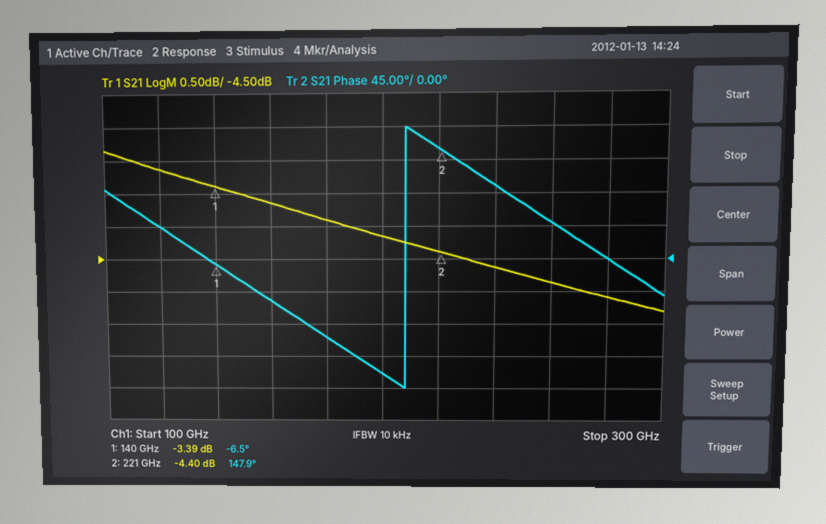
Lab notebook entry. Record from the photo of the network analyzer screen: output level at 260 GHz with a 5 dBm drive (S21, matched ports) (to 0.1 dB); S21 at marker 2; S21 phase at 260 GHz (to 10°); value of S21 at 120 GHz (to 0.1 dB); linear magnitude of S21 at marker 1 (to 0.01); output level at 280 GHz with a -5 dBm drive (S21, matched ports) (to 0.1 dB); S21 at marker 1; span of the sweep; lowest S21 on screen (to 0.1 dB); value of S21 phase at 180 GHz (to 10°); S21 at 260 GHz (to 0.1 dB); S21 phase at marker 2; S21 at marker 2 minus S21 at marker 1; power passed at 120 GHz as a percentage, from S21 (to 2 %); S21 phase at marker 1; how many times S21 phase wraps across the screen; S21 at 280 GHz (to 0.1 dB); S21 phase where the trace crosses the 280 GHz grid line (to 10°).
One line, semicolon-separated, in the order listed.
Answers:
0.1 dBm; -4.40 dB; 50°; -3.1 dB; 0.68; -10.1 dBm; -3.39 dB; 200 GHz; -5.3 dB; -110°; -4.9 dB; 147.9°; -1.01 dB; 48 %; -6.5°; 1; -5.1 dB; 0°
